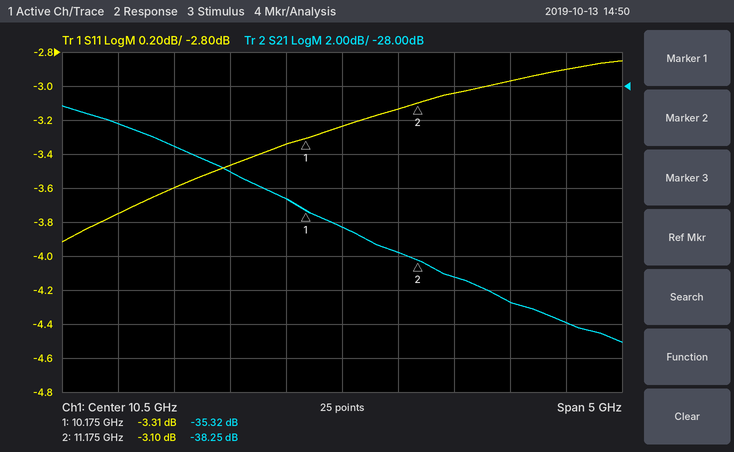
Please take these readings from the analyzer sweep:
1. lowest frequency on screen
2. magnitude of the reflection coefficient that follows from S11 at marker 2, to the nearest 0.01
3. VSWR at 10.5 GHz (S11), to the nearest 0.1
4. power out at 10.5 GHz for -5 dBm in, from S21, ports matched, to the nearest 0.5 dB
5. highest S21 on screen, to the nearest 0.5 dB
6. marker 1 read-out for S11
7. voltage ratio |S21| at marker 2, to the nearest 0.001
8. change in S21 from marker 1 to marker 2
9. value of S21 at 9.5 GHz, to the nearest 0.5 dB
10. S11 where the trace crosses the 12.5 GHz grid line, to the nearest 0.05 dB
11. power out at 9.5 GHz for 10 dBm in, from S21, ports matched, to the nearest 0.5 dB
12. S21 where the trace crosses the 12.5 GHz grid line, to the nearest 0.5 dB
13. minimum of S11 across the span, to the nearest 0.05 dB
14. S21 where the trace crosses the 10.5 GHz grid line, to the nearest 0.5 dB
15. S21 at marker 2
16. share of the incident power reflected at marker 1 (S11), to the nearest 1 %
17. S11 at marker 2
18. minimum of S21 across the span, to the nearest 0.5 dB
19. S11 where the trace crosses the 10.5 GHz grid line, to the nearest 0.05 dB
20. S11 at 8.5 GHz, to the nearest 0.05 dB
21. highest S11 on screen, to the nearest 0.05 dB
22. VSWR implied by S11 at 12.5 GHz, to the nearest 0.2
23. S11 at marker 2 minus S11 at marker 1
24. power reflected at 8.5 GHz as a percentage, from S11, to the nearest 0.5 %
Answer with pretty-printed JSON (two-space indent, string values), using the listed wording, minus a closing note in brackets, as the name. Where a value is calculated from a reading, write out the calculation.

{
  "lowest frequency on screen": "8 GHz",
  "magnitude of the reflection coefficient that follows from S11 at marker 2, to the nearest 0.01": "10^(-3.1/20) ≈ 0.70",
  "VSWR at 10.5 GHz (S11), to the nearest 0.1": "|Γ| = 10^(-3.25/20) = 0.6879; VSWR = (1 + 0.6879)/(1 − 0.6879) ≈ 5.4",
  "power out at 10.5 GHz for -5 dBm in, from S21, ports matched, to the nearest 0.5 dB": "-5 dBm + (-36.5 dB) = -41.5 dBm",
  "highest S21 on screen, to the nearest 0.5 dB": "-29.0 dB",
  "marker 1 read-out for S11": "-3.31 dB",
  "voltage ratio |S21| at marker 2, to the nearest 0.001": "10^(-38.25/20) ≈ 0.012",
  "change in S21 from marker 1 to marker 2": "-38.25 − (-35.32) = -2.93 dB",
  "value of S21 at 9.5 GHz, to the nearest 0.5 dB": "-33.0 dB",
  "S11 where the trace crosses the 12.5 GHz grid line, to the nearest 0.05 dB": "-2.90 dB",
  "power out at 9.5 GHz for 10 dBm in, from S21, ports matched, to the nearest 0.5 dB": "10 dBm + (-33.0 dB) = -23.0 dBm",
  "S21 where the trace crosses the 12.5 GHz grid line, to the nearest 0.5 dB": "-42.0 dB",
  "minimum of S11 across the span, to the nearest 0.05 dB": "-3.90 dB",
  "S21 where the trace crosses the 10.5 GHz grid line, to the nearest 0.5 dB": "-36.5 dB",
  "S21 at marker 2": "-38.25 dB",
  "share of the incident power reflected at marker 1 (S11), to the nearest 1 %": "10^(-3.31/10) ≈ 47 %",
  "S11 at marker 2": "-3.10 dB",
  "minimum of S21 across the span, to the nearest 0.5 dB": "-43.0 dB",
  "S11 where the trace crosses the 10.5 GHz grid line, to the nearest 0.05 dB": "-3.25 dB",
  "S11 at 8.5 GHz, to the nearest 0.05 dB": "-3.75 dB",
  "highest S11 on screen, to the nearest 0.05 dB": "-2.85 dB",
  "VSWR implied by S11 at 12.5 GHz, to the nearest 0.2": "|Γ| = 10^(-2.9/20) = 0.7161; VSWR = (1 + 0.7161)/(1 − 0.7161) ≈ 6.0",
  "S11 at marker 2 minus S11 at marker 1": "-3.1 − (-3.31) = 0.21 dB",
  "power reflected at 8.5 GHz as a percentage, from S11, to the nearest 0.5 %": "10^(-3.75/10) ≈ 42.2 %, so 42.0 % to the nearest 0.5 %"
}
